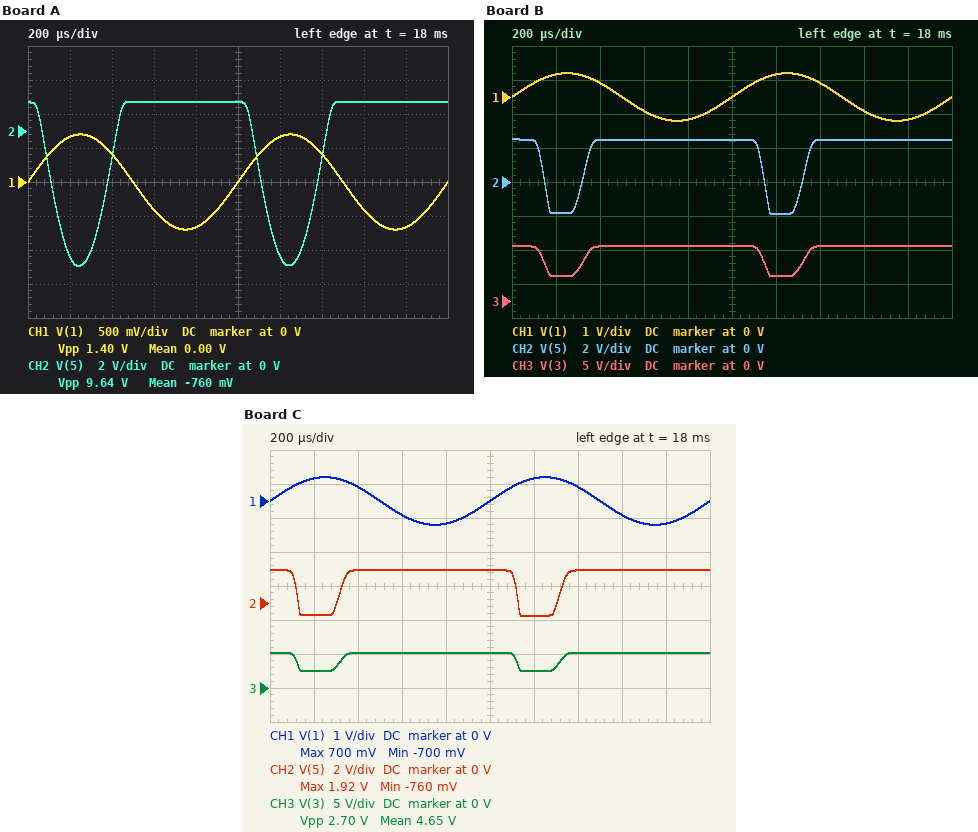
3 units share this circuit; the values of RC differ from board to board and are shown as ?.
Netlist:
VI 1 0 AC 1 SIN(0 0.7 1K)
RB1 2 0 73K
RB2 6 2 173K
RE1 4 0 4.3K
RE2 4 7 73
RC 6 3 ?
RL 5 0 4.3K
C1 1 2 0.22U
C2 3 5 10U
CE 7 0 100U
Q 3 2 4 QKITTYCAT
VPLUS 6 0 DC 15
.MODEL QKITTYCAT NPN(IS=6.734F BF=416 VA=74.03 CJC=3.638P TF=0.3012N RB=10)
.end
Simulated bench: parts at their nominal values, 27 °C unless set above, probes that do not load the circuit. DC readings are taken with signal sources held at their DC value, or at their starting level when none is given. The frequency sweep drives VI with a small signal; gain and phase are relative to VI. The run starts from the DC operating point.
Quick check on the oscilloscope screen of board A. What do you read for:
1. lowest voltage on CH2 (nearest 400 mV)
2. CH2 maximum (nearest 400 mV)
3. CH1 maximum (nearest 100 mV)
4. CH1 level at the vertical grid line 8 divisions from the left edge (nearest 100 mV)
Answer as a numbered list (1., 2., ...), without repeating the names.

1. -8.0 V
2. 1.6 V
3. 700 mV
4. -400 mV
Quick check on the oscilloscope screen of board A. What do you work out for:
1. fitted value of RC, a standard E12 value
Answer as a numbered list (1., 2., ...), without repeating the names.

1. 2.7 kΩ
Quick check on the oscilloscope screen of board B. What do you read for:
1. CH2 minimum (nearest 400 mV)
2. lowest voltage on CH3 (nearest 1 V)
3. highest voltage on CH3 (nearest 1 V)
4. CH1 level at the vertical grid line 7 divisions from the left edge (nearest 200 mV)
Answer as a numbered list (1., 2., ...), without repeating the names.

1. -2.0 V
2. 4 V
3. 8 V
4. 400 mV
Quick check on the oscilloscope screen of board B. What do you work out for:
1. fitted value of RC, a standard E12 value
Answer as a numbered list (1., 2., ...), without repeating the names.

1. 12 kΩ
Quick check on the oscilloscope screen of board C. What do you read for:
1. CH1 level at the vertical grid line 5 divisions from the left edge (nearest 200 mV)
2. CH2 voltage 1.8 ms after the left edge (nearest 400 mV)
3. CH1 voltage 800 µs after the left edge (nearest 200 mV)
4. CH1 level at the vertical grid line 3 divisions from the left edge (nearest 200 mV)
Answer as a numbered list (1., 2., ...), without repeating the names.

1. 0 V
2. 2.0 V
3. -600 mV
4. -400 mV
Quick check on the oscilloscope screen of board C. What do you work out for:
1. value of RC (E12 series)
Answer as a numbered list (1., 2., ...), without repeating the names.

1. 22 kΩ
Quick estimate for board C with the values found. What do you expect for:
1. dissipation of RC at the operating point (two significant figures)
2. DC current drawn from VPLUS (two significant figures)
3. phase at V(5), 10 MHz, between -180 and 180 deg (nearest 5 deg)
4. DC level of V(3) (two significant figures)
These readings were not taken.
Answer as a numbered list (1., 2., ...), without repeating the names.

1. 7.0 mW
2. 630 µA
3. 165 deg
4. 2.6 V
